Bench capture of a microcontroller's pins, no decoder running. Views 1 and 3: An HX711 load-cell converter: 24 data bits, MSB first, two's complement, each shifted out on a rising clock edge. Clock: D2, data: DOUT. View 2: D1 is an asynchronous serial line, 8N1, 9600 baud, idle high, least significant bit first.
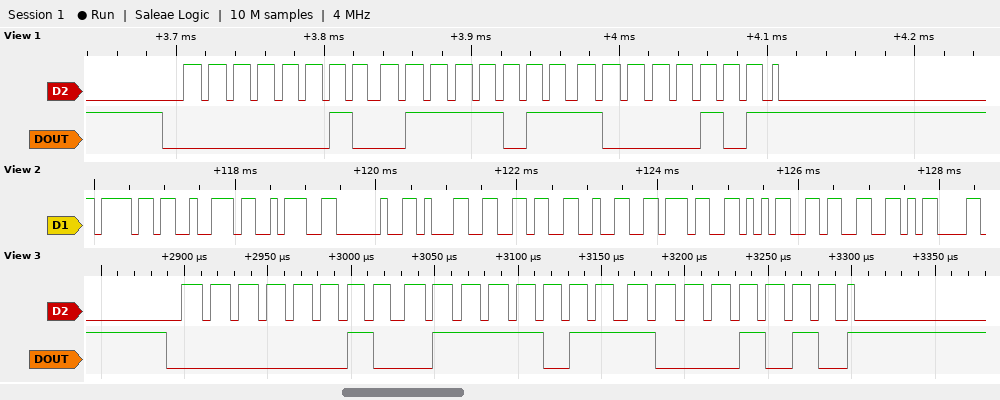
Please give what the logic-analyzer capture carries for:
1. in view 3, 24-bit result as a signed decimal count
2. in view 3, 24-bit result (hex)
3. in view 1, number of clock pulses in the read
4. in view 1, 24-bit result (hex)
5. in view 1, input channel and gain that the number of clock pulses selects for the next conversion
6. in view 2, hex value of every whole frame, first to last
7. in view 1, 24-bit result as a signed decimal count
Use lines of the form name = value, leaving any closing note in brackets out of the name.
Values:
in view 3, 24-bit result as a signed decimal count = 162698
in view 3, 24-bit result = 0x027B8A
in view 1, number of clock pulses in the read = 25
in view 1, 24-bit result = 0x027B85
in view 1, input channel and gain that the number of clock pulses selects for the next conversion = channel A, gain 128
in view 2, hex value of every whole frame, first to last = 6F 72 3A 20 31 36 32 37 35 33 0D
in view 1, 24-bit result as a signed decimal count = 162693
